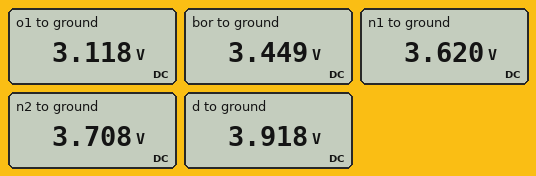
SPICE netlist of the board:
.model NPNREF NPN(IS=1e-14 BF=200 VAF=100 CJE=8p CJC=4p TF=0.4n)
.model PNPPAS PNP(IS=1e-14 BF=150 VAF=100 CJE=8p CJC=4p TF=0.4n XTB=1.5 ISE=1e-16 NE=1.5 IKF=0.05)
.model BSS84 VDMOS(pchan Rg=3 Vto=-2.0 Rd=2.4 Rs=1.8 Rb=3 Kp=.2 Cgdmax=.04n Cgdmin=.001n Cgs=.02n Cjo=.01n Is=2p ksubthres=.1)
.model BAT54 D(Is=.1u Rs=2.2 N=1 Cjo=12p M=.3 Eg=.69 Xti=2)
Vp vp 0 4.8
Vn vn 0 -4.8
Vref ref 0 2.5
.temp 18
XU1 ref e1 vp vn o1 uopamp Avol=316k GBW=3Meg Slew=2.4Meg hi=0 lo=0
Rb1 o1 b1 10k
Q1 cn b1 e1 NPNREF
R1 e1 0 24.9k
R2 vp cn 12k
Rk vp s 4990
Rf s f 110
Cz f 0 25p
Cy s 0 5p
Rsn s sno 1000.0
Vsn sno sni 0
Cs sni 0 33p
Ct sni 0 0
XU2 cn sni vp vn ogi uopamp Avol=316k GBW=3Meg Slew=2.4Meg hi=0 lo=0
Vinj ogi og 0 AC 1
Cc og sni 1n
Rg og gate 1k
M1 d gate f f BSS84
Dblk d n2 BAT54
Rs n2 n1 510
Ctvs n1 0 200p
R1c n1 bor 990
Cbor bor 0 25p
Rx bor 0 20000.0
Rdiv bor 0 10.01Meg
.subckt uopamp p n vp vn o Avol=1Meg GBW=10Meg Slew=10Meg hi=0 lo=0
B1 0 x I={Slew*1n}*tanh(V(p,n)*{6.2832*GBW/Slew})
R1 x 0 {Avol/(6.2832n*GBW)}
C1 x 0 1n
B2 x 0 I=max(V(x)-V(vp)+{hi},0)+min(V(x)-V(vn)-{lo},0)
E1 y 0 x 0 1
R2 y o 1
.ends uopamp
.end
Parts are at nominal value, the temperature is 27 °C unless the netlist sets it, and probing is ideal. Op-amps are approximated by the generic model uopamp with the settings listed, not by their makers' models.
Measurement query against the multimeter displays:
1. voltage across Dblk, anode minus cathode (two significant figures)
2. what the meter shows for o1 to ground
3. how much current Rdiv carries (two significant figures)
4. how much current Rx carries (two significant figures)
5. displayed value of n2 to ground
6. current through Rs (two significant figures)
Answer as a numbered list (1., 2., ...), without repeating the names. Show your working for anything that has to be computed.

1. 3.918 V - 3.708 V = 210 mV
2. 3.118 V
3. (3.449 V) / 10.01 MΩ = 340 nA
4. (3.449 V) / 20 kΩ = 170 µA
5. 3.708 V
6. (3.708 V - 3.62 V) / 510 Ω = 170 µA
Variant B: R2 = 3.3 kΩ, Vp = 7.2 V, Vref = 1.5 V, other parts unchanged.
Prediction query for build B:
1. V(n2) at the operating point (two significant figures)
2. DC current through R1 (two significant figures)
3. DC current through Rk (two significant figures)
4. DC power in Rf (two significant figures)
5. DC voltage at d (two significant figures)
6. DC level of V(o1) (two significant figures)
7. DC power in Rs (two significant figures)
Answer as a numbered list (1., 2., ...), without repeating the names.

1. 850 mV
2. 60 µA
3. 40 µA
4. 170 nW
5. 1.0 V
6. 2.1 V
7. 800 nW
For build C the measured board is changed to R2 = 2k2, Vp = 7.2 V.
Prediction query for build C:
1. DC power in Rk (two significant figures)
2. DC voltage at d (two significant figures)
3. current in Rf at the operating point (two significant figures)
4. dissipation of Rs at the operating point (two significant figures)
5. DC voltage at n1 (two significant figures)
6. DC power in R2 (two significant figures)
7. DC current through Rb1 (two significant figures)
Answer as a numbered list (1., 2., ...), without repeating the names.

1. 9.7 µW
2. 1.1 V
3. 44 µA
4. 990 nW
5. 920 mV
6. 22 µW
7. 480 nA
